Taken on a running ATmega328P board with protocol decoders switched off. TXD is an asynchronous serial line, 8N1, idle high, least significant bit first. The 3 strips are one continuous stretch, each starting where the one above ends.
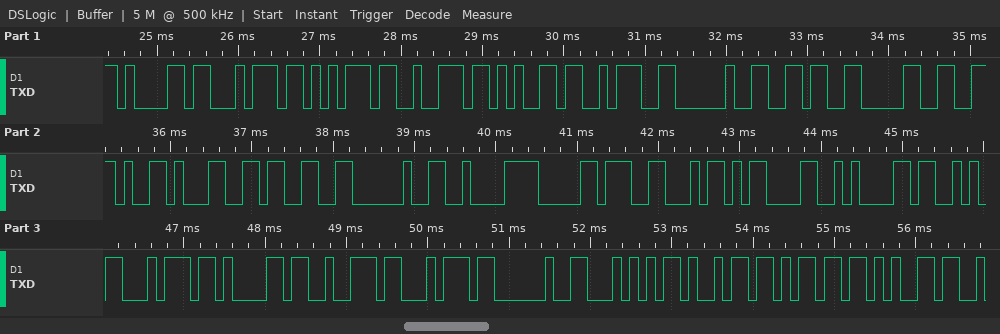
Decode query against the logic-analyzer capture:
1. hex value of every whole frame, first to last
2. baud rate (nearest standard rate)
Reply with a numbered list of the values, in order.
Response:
1. 0x61 0x74 0x75 0x72 0x65 0x3A 0x20 0x36 0x30 0x2E 0x31 0x33 0x20 0xC2 0xB0 0x46 0x0D 0x0A 0x53 0x74 0x61 0x72 0x74 0x20 0x54 0x69 0x6D 0x65
2. 9600 baud
